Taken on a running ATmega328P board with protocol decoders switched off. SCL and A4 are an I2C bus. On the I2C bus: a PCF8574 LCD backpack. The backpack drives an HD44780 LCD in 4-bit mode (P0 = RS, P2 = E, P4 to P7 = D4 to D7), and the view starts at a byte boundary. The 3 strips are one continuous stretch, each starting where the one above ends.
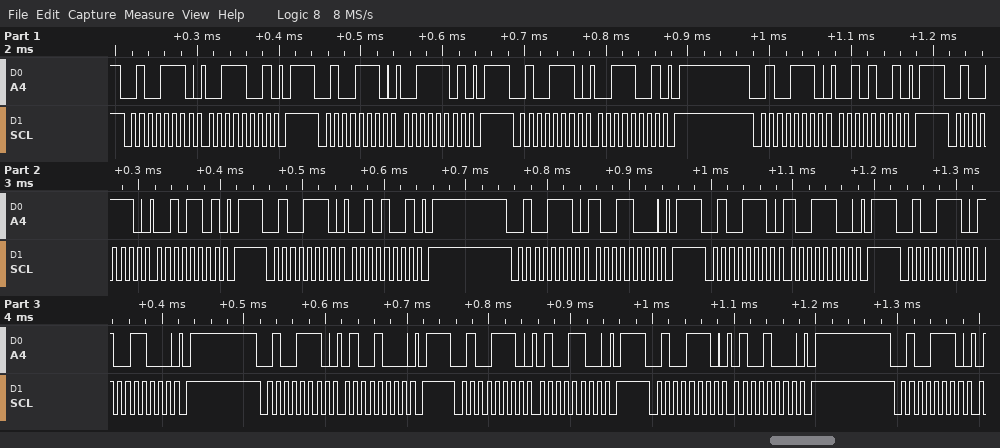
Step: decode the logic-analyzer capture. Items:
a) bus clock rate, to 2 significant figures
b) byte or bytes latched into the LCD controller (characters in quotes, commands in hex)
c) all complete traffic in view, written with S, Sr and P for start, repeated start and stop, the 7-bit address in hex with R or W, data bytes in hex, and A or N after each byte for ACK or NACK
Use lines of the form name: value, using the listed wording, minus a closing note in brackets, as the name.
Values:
bus clock rate, to 2 significant figures: 100 kHz
byte or bytes latched into the LCD controller: '2' 0x94
all complete traffic in view, written with S, Sr and P for start, repeated start and stop, the 7-bit address in hex with R or W, data bytes in hex, and A or N after each byte for ACK or NACK: S 27W A 39 A P S 27W A 3D A P S 27W A 39 A P S 27W A 29 A P S 27W A 2D A P S 27W A 29 A P S 27W A 98 A P S 27W A 9C A P S 27W A 98 A P S 27W A 48 A P S 27W A 4C A P S 27W A 48 A P S 27W A
